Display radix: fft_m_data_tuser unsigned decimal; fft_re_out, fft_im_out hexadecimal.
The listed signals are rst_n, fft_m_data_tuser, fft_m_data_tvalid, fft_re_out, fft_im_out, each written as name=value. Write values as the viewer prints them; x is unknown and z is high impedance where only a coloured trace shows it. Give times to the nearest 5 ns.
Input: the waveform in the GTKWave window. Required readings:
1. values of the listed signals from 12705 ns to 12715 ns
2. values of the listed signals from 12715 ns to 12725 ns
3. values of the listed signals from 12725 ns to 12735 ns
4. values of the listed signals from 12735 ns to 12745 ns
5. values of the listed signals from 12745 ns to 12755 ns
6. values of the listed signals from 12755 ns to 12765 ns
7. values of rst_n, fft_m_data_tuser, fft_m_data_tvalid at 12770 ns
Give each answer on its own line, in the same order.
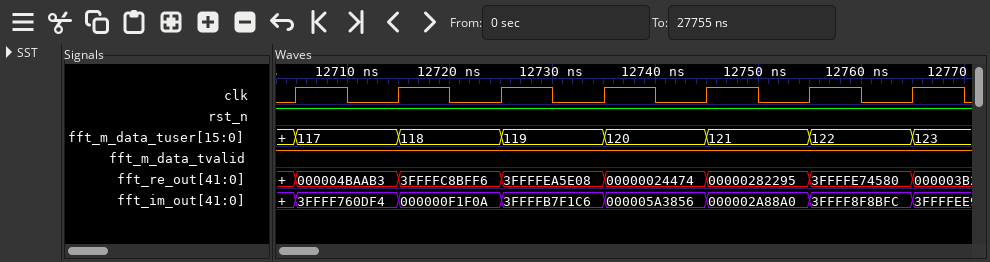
rst_n=1, fft_m_data_tuser=117, fft_m_data_tvalid=1, fft_re_out=000004BAAB3, fft_im_out=3FFFF760DF4
rst_n=1, fft_m_data_tuser=118, fft_m_data_tvalid=1, fft_re_out=3FFFFC8BFF6, fft_im_out=000000F1F0A
rst_n=1, fft_m_data_tuser=119, fft_m_data_tvalid=1, fft_re_out=3FFFFEA5E08, fft_im_out=3FFFFB7F1C6
rst_n=1, fft_m_data_tuser=120, fft_m_data_tvalid=1, fft_re_out=00000024474, fft_im_out=000005A3856
rst_n=1, fft_m_data_tuser=121, fft_m_data_tvalid=1, fft_re_out=00000282295, fft_im_out=000002A88A0
rst_n=1, fft_m_data_tuser=122, fft_m_data_tvalid=1, fft_re_out=3FFFFE74580, fft_im_out=3FFFF8F8BFC
rst_n=1, fft_m_data_tuser=123, fft_m_data_tvalid=1
